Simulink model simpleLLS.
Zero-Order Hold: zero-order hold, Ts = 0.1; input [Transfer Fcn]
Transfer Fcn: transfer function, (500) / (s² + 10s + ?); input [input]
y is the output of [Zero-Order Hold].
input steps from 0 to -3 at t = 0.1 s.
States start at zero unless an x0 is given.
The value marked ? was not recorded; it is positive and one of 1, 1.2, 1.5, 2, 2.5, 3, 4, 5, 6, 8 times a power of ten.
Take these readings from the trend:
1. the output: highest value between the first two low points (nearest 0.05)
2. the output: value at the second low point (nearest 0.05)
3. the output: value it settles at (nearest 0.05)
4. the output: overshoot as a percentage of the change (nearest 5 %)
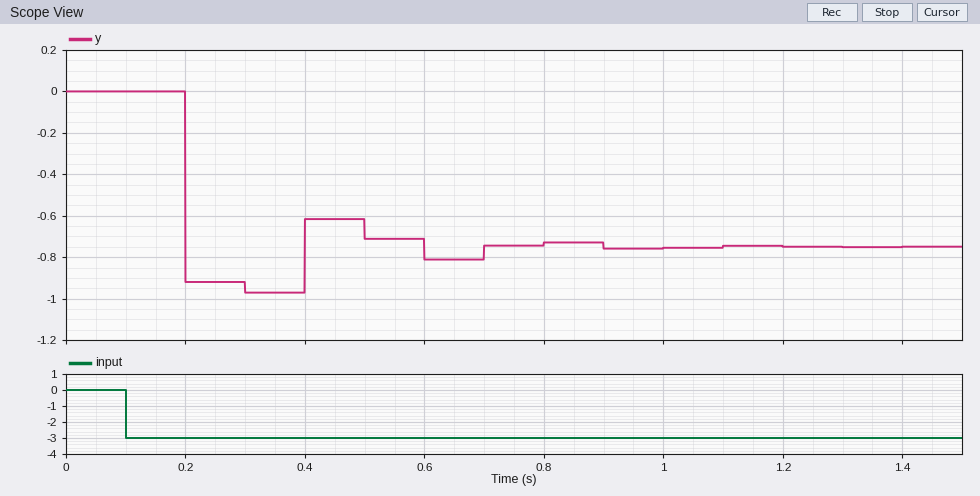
-0.60
-0.80
-0.75
30 %
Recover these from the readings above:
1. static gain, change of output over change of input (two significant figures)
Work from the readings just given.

0.25
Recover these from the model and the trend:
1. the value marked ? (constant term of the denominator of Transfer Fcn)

2000
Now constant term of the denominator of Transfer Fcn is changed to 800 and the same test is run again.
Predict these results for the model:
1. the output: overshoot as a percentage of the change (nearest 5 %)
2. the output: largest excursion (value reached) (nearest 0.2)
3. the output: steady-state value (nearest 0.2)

55 %
-2.8
-1.8
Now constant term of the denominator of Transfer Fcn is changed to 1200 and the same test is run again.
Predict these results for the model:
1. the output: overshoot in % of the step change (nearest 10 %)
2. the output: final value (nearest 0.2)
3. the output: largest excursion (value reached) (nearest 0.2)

60 %
-1.2
-2.0
